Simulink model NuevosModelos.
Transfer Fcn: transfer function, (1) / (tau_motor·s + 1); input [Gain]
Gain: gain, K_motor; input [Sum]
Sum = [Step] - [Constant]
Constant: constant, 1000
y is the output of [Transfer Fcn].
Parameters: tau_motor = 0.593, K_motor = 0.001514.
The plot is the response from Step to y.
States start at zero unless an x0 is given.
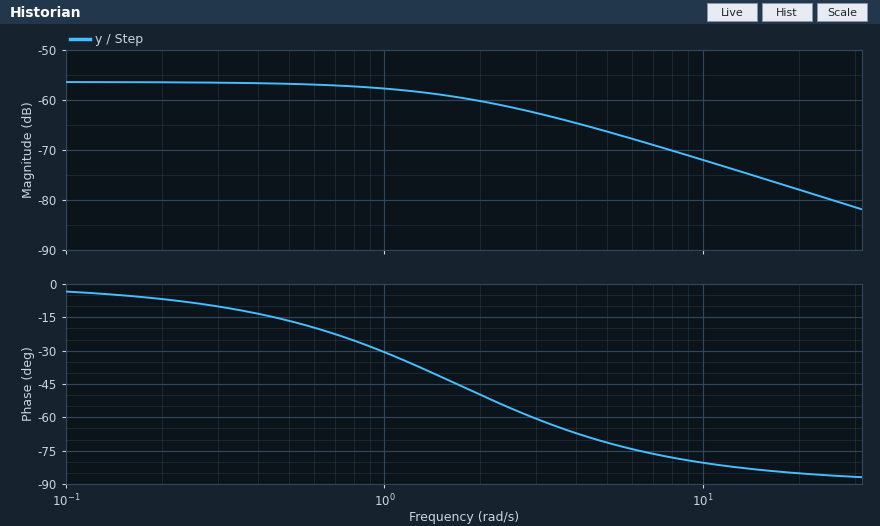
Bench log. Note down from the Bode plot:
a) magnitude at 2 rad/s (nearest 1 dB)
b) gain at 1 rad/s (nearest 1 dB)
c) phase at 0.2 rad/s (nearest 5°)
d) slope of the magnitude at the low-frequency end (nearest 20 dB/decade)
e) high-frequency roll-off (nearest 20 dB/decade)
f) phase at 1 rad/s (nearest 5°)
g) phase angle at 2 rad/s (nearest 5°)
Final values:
-60 dB
-58 dB
-5°
0 dB/decade
-20 dB/decade
-30°
-50°
